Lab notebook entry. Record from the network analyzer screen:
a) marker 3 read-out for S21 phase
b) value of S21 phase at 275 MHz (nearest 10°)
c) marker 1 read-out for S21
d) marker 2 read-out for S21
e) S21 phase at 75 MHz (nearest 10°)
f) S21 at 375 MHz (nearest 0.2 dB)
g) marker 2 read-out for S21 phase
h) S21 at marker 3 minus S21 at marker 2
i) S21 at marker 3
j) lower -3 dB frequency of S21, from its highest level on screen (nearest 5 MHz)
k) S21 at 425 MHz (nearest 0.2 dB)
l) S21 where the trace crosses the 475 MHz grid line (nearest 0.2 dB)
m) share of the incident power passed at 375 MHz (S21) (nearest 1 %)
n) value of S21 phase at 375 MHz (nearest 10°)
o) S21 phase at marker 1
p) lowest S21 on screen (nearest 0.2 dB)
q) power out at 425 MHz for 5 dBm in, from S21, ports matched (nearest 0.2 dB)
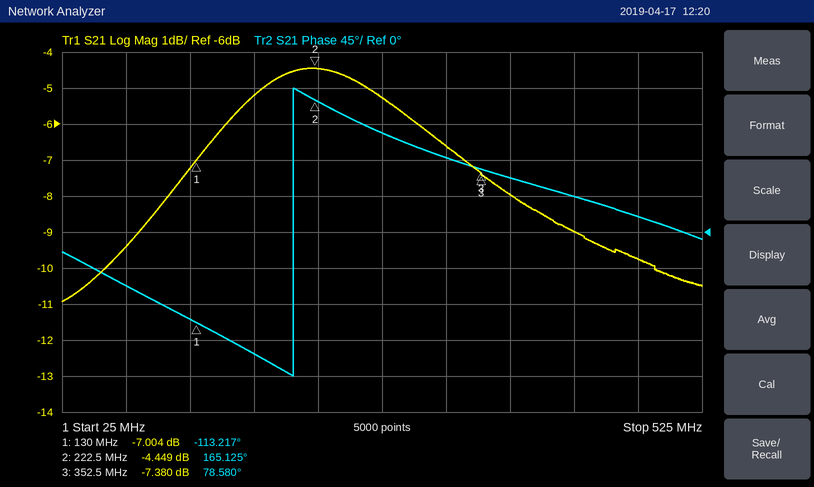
78.580°
120°
-7.004 dB
-4.449 dB
-70°
-8.0 dB
165.125°
-2.931 dB
-7.380 dB
120 MHz
-9.0 dB
-9.8 dB
16 %
70°
-113.217°
-11.0 dB
-4.0 dBm
